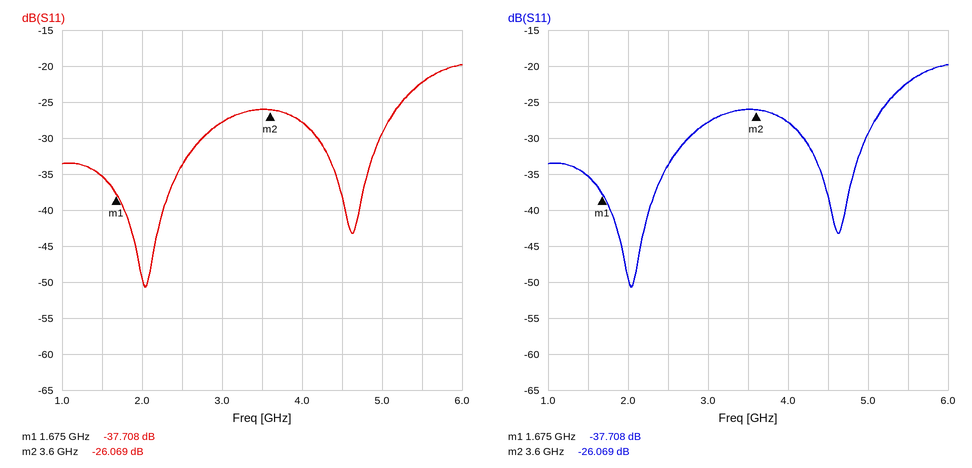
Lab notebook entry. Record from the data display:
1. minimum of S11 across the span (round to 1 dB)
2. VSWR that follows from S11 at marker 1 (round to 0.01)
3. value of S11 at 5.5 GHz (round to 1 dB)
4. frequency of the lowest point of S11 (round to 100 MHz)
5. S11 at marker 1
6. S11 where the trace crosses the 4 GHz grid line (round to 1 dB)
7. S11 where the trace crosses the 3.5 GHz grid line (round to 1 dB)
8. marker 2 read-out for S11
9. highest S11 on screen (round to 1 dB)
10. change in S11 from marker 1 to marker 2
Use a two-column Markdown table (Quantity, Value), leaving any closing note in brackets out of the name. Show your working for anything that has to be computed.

| Quantity | Value |
|---|---|
| minimum of S11 across the span | -51 dB |
| VSWR that follows from S11 at marker 1 | (1 + 0.0130)/(1 − 0.0130) ≈ 1.03 |
| value of S11 at 5.5 GHz | -22 dB |
| frequency of the lowest point of S11 | 2.0 GHz |
| S11 at marker 1 | -37.708 dB |
| S11 where the trace crosses the 4 GHz grid line | -28 dB |
| S11 where the trace crosses the 3.5 GHz grid line | -26 dB |
| marker 2 read-out for S11 | -26.069 dB |
| highest S11 on screen | -20 dB |
| change in S11 from marker 1 to marker 2 | -26.069 − (-37.708) = 11.639 dB |
